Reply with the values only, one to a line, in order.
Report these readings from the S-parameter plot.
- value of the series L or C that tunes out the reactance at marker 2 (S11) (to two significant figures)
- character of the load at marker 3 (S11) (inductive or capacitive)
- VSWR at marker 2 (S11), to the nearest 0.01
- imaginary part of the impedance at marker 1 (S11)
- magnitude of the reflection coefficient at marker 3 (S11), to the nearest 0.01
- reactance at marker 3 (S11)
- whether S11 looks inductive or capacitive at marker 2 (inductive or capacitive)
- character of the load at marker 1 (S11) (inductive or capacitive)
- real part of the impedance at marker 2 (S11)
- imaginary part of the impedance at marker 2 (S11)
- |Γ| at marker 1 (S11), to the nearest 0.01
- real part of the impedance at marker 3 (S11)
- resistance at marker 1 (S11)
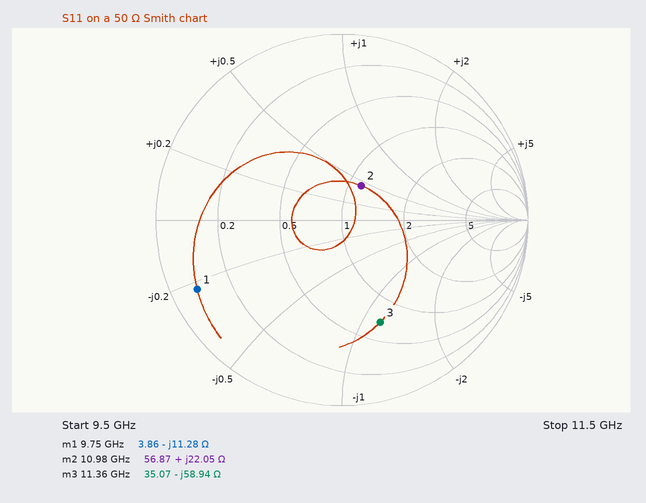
660 fF
capacitive
1.54
-11.28 Ω
0.59
-58.94 Ω
inductive
capacitive
56.87 Ω
+22.05 Ω
0.86
35.07 Ω
3.86 Ω
